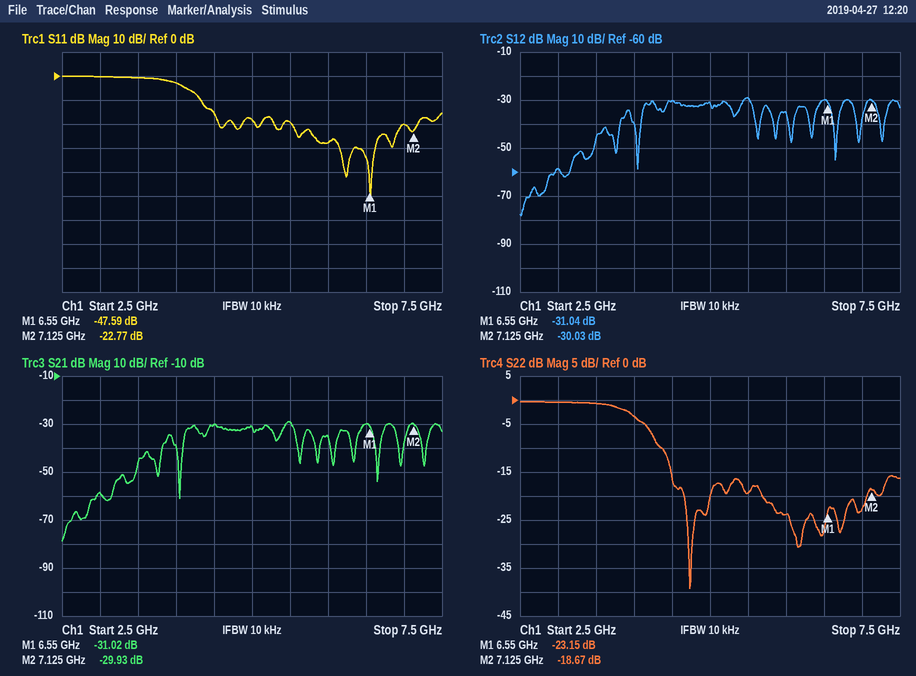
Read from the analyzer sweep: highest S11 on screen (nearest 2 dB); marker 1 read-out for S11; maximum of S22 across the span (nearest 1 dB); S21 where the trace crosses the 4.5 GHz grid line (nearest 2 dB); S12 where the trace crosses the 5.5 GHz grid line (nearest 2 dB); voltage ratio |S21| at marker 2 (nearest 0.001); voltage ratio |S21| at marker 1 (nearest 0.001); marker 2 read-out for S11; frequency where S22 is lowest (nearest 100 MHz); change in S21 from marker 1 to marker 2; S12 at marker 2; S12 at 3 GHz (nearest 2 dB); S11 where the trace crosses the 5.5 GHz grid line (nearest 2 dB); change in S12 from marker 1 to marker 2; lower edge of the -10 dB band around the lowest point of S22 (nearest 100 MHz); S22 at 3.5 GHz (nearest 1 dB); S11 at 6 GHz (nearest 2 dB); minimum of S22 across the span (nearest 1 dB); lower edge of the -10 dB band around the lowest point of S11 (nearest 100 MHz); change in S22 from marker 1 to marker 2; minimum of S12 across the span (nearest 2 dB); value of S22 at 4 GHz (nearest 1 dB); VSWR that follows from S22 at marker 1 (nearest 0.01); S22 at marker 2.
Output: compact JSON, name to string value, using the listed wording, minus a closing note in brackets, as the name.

{"highest S11 on screen": "0 dB", "marker 1 read-out for S11": "-47.59 dB", "maximum of S22 across the span": "0 dB", "S21 where the trace crosses the 4.5 GHz grid line": "-30 dB", "S12 where the trace crosses the 5.5 GHz grid line": "-30 dB", "voltage ratio |S21| at marker 2": "0.032", "voltage ratio |S21| at marker 1": "0.028", "marker 2 read-out for S11": "-22.77 dB", "frequency where S22 is lowest": "4.7 GHz", "change in S21 from marker 1 to marker 2": "1.09 dB", "S12 at marker 2": "-30.03 dB", "S12 at 3 GHz": "-58 dB", "S11 where the trace crosses the 5.5 GHz grid line": "-20 dB", "change in S12 from marker 1 to marker 2": "1.01 dB", "lower edge of the -10 dB band around the lowest point of S22": "4.4 GHz", "S22 at 3.5 GHz": "-1 dB", "S11 at 6 GHz": "-28 dB", "minimum of S22 across the span": "-39 dB", "lower edge of the -10 dB band around the lowest point of S11": "4.3 GHz", "change in S22 from marker 1 to marker 2": "4.48 dB", "minimum of S12 across the span": "-78 dB", "value of S22 at 4 GHz": "-3 dB", "VSWR that follows from S22 at marker 1": "1.15", "S22 at marker 2": "-18.67 dB"}
